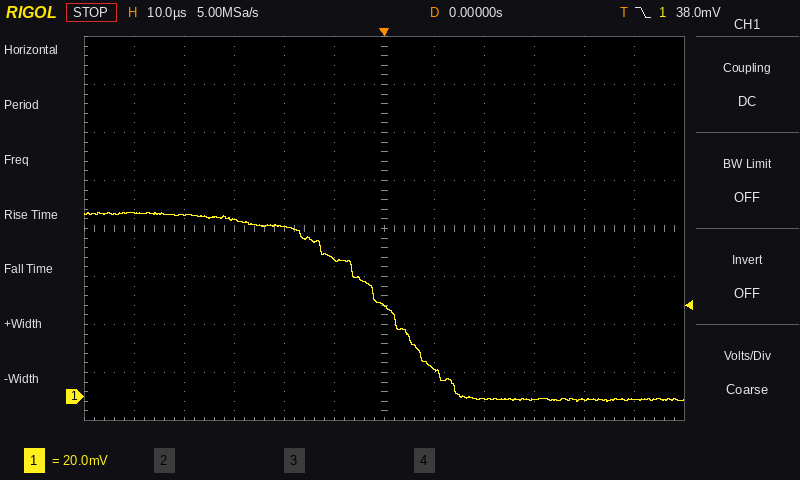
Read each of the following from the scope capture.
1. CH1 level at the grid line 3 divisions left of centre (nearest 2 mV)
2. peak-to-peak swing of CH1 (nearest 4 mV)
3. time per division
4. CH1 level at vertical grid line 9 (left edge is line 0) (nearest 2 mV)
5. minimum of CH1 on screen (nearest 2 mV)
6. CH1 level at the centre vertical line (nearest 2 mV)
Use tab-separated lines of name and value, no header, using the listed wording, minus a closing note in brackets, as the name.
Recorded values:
CH1 level at the grid line 3 divisions left of centre	74 mV
peak-to-peak swing of CH1	80 mV
time per division	10 µs
CH1 level at vertical grid line 9 (left edge is line 0)	-2 mV
minimum of CH1 on screen	-2 mV
CH1 level at the centre vertical line	38 mV
